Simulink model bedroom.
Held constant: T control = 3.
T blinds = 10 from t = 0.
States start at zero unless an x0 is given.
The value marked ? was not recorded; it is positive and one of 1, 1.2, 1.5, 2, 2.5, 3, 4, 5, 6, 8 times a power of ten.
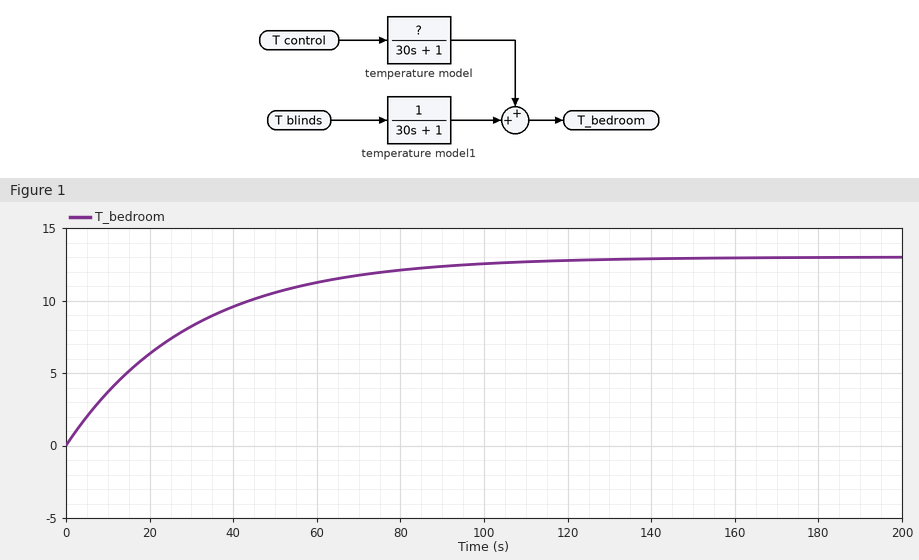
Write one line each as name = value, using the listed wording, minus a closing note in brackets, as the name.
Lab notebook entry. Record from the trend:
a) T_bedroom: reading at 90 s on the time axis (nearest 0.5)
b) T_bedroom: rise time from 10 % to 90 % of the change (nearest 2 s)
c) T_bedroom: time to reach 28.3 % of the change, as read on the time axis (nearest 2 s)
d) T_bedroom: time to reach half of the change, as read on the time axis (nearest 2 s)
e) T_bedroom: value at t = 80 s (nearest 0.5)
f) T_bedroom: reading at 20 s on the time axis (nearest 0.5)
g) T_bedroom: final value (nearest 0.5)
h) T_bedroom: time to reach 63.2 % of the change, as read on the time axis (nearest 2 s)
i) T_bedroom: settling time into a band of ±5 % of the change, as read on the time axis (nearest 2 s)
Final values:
T_bedroom: reading at 90 s on the time axis = 12.5
T_bedroom: rise time from 10 % to 90 % of the change = 66 s
T_bedroom: time to reach 28.3 % of the change, as read on the time axis = 10 s
T_bedroom: time to reach half of the change, as read on the time axis = 20 s
T_bedroom: value at t = 80 s = 12.0
T_bedroom: reading at 20 s on the time axis = 6.5
T_bedroom: final value = 13.0
T_bedroom: time to reach 63.2 % of the change, as read on the time axis = 30 s
T_bedroom: settling time into a band of ±5 % of the change, as read on the time axis = 90 s
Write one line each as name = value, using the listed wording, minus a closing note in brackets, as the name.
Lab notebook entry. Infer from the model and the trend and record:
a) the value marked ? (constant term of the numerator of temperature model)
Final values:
the value marked ? = 1
